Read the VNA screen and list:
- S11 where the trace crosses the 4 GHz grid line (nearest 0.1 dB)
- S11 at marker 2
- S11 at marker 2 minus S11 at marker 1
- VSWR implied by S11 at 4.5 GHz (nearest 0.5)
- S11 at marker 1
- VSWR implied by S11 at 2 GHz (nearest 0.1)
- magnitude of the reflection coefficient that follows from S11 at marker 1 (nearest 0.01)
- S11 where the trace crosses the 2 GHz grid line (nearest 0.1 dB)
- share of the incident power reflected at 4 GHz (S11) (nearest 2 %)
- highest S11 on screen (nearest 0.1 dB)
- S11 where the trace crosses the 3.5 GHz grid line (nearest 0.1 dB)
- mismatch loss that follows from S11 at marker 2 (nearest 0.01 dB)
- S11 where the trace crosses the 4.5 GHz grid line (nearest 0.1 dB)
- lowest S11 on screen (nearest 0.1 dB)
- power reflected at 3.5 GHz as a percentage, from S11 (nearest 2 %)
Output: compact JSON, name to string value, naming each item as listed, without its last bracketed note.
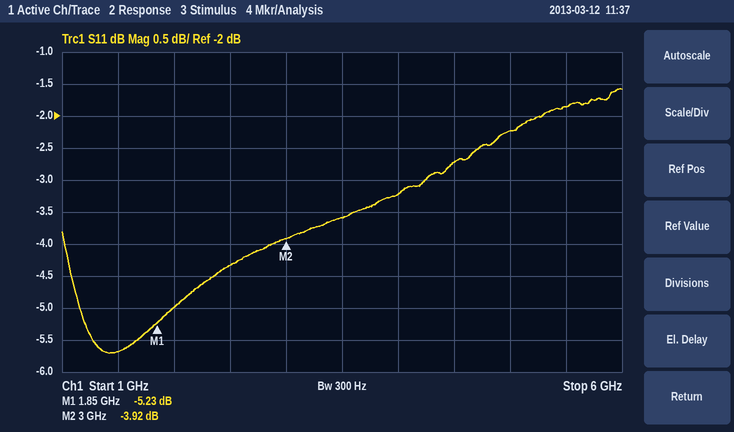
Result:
{"S11 where the trace crosses the 4 GHz grid line": "-3.2 dB", "S11 at marker 2": "-3.92 dB", "S11 at marker 2 minus S11 at marker 1": "1.31 dB", "VSWR implied by S11 at 4.5 GHz": "6.5", "S11 at marker 1": "-5.23 dB", "VSWR implied by S11 at 2 GHz": "3.6", "magnitude of the reflection coefficient that follows from S11 at marker 1": "0.55", "S11 where the trace crosses the 2 GHz grid line": "-5.0 dB", "share of the incident power reflected at 4 GHz (S11)": "48 %", "highest S11 on screen": "-1.6 dB", "S11 where the trace crosses the 3.5 GHz grid line": "-3.6 dB", "mismatch loss that follows from S11 at marker 2": "2.26 dB", "S11 where the trace crosses the 4.5 GHz grid line": "-2.7 dB", "lowest S11 on screen": "-5.7 dB", "power reflected at 3.5 GHz as a percentage, from S11": "44 %"}
